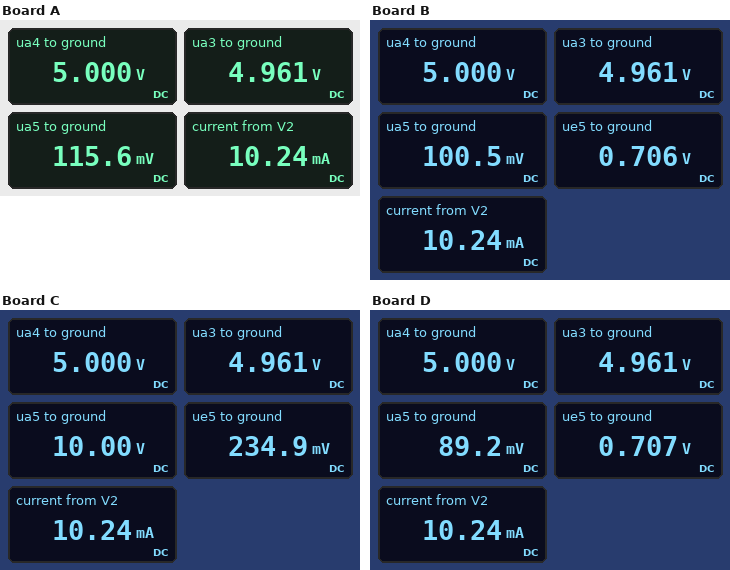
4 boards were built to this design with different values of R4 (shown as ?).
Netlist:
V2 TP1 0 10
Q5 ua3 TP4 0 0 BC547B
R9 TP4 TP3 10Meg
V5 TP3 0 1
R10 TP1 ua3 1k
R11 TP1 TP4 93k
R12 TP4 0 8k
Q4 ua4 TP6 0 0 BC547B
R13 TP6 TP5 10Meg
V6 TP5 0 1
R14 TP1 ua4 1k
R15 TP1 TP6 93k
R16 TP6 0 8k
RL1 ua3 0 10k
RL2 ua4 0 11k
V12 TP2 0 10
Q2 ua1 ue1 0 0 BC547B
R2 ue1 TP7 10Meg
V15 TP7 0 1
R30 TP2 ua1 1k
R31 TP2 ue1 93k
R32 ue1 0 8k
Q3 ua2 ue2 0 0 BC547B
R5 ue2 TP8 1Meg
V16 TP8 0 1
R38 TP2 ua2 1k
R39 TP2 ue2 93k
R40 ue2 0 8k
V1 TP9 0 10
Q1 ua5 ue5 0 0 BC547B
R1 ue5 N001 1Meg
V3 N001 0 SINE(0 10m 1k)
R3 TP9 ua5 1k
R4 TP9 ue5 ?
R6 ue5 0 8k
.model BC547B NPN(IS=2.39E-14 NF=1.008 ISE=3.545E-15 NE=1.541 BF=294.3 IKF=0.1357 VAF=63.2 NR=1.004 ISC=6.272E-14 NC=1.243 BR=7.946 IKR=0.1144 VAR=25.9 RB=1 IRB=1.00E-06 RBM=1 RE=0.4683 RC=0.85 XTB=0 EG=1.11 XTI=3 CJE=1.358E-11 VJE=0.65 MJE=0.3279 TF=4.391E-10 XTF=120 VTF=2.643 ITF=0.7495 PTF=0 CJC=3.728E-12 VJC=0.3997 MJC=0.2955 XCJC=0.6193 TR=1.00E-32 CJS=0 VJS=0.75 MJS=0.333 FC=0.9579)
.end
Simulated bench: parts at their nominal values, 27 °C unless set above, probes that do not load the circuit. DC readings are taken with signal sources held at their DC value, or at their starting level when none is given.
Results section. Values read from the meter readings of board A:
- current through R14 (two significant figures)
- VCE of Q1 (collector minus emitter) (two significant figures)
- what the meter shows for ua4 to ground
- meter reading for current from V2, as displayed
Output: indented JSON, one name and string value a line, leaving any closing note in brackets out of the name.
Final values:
{
  "current through R14": "5.0 mA",
  "VCE of Q1 (collector minus emitter)": "120 mV",
  "what the meter shows for ua4 to ground": "5.000 V",
  "meter reading for current from V2, as displayed": "10.24 mA"
}
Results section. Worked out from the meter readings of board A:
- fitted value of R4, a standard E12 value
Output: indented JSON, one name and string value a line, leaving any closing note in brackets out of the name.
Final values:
{
  "fitted value of R4, a standard E12 value": "56 kΩ"
}
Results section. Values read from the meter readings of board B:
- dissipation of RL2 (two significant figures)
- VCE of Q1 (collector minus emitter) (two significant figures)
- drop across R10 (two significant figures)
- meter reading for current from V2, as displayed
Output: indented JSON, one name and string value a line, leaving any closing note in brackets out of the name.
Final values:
{
  "dissipation of RL2": "2.3 mW",
  "VCE of Q1 (collector minus emitter)": "100 mV",
  "drop across R10": "5.0 V",
  "meter reading for current from V2, as displayed": "10.24 mA"
}
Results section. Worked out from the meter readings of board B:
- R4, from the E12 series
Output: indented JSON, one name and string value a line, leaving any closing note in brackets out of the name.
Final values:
{
  "R4, from the E12 series": "47 kΩ"
}
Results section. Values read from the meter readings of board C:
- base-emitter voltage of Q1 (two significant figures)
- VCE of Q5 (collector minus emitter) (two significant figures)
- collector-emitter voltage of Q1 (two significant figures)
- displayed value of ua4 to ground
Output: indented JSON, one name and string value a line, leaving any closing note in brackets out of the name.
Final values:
{
  "base-emitter voltage of Q1": "230 mV",
  "VCE of Q5 (collector minus emitter)": "5.0 V",
  "collector-emitter voltage of Q1": "10 V",
  "displayed value of ua4 to ground": "5.000 V"
}
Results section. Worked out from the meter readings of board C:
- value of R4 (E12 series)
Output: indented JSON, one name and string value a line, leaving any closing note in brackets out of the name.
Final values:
{
  "value of R4": "330 kΩ"
}
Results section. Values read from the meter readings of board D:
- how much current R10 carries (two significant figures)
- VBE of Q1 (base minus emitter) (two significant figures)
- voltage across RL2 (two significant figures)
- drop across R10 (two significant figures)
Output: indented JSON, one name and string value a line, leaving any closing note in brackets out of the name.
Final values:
{
  "how much current R10 carries": "5.0 mA",
  "VBE of Q1 (base minus emitter)": "710 mV",
  "voltage across RL2": "5.0 V",
  "drop across R10": "5.0 V"
}
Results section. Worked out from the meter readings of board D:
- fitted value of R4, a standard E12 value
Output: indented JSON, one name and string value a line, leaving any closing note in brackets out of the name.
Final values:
{
  "fitted value of R4, a standard E12 value": "39 kΩ"
}
